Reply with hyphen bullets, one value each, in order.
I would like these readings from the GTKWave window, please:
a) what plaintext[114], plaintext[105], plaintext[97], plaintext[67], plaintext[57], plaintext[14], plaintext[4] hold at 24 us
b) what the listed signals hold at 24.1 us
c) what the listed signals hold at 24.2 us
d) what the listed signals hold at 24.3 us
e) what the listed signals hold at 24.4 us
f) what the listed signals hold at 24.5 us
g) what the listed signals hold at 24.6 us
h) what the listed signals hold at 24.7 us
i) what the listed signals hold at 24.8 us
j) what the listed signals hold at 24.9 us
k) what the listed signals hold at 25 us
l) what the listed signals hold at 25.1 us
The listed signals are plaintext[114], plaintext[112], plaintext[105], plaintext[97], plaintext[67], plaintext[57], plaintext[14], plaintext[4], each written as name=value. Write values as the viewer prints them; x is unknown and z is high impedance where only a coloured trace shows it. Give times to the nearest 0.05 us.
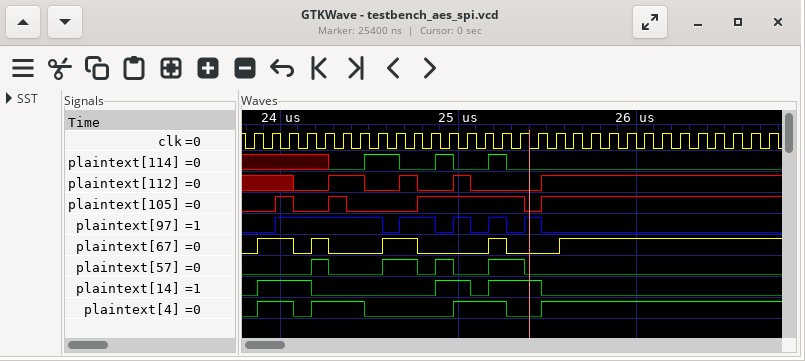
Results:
- plaintext[114]=x, plaintext[105]=1, plaintext[97]=1, plaintext[67]=1, plaintext[57]=0, plaintext[14]=1, plaintext[4]=1
- plaintext[114]=x, plaintext[112]=0, plaintext[105]=0, plaintext[97]=1, plaintext[67]=0, plaintext[57]=0, plaintext[14]=1, plaintext[4]=0
- plaintext[114]=x, plaintext[112]=0, plaintext[105]=0, plaintext[97]=1, plaintext[67]=1, plaintext[57]=1, plaintext[14]=0, plaintext[4]=1
- plaintext[114]=0, plaintext[112]=1, plaintext[105]=1, plaintext[97]=1, plaintext[67]=0, plaintext[57]=0, plaintext[14]=0, plaintext[4]=1
- plaintext[114]=0, plaintext[112]=1, plaintext[105]=0, plaintext[97]=1, plaintext[67]=0, plaintext[57]=0, plaintext[14]=0, plaintext[4]=1
- plaintext[114]=1, plaintext[112]=0, plaintext[105]=0, plaintext[97]=1, plaintext[67]=0, plaintext[57]=0, plaintext[14]=0, plaintext[4]=0
- plaintext[114]=1, plaintext[112]=0, plaintext[105]=0, plaintext[97]=0, plaintext[67]=1, plaintext[57]=1, plaintext[14]=0, plaintext[4]=0
- plaintext[114]=0, plaintext[112]=1, plaintext[105]=0, plaintext[97]=1, plaintext[67]=1, plaintext[57]=1, plaintext[14]=0, plaintext[4]=0
- plaintext[114]=0, plaintext[112]=0, plaintext[105]=1, plaintext[97]=1, plaintext[67]=0, plaintext[57]=0, plaintext[14]=0, plaintext[4]=0
- plaintext[114]=1, plaintext[112]=0, plaintext[105]=1, plaintext[97]=0, plaintext[67]=0, plaintext[57]=1, plaintext[14]=1, plaintext[4]=0
- plaintext[114]=0, plaintext[112]=1, plaintext[105]=1, plaintext[97]=1, plaintext[67]=0, plaintext[57]=0, plaintext[14]=1, plaintext[4]=1
- plaintext[114]=0, plaintext[112]=0, plaintext[105]=1, plaintext[97]=0, plaintext[67]=0, plaintext[57]=0, plaintext[14]=0, plaintext[4]=1
